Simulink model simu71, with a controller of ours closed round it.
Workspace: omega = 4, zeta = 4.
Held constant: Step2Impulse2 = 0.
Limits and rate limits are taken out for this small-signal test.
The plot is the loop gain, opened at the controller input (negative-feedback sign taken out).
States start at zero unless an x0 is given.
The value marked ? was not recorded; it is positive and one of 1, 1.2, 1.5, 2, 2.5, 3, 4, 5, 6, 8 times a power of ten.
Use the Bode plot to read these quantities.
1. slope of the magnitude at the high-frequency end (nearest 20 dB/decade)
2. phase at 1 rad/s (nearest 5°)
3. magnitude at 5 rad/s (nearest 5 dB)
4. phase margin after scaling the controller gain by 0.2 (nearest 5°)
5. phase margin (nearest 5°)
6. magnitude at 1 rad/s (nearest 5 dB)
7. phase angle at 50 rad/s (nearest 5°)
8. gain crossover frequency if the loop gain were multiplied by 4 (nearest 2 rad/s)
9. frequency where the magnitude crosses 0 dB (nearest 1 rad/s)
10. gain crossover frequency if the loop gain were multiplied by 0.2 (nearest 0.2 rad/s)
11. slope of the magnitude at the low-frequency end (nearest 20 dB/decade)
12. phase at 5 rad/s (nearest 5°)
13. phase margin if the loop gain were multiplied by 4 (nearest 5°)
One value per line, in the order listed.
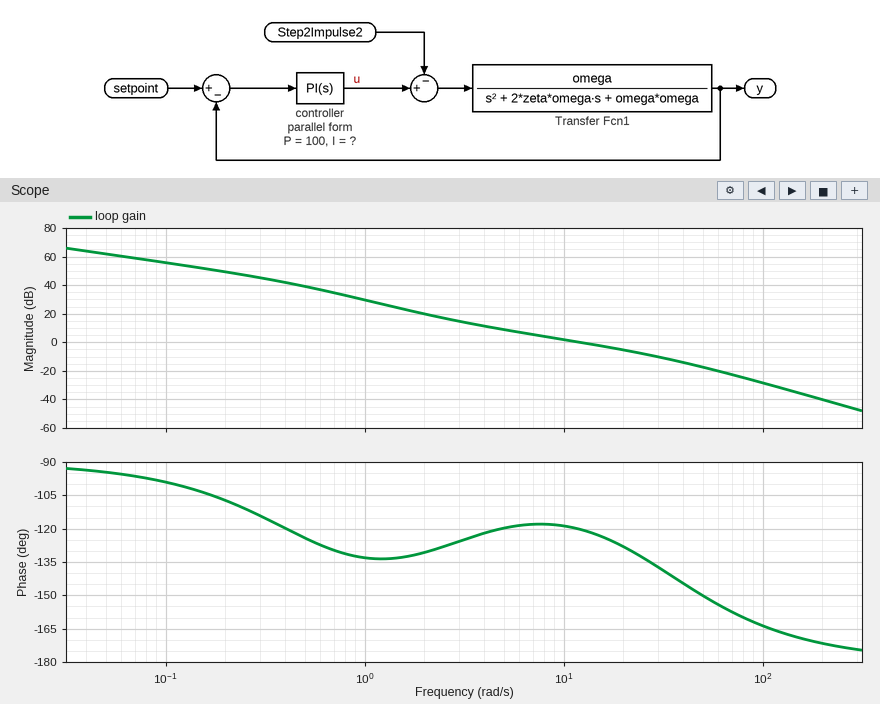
-40 dB/decade
-135°
10 dB
55°
60°
30 dB
-150°
34 rad/s
12 rad/s
3.2 rad/s
-20 dB/decade
-120°
40°
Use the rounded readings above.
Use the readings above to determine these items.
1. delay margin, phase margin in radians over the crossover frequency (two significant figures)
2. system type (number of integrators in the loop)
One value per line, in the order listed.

0.087 s
1
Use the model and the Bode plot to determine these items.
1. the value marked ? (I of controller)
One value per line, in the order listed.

250
